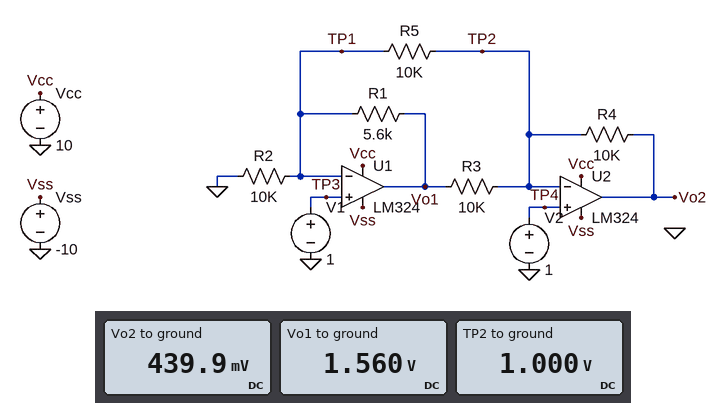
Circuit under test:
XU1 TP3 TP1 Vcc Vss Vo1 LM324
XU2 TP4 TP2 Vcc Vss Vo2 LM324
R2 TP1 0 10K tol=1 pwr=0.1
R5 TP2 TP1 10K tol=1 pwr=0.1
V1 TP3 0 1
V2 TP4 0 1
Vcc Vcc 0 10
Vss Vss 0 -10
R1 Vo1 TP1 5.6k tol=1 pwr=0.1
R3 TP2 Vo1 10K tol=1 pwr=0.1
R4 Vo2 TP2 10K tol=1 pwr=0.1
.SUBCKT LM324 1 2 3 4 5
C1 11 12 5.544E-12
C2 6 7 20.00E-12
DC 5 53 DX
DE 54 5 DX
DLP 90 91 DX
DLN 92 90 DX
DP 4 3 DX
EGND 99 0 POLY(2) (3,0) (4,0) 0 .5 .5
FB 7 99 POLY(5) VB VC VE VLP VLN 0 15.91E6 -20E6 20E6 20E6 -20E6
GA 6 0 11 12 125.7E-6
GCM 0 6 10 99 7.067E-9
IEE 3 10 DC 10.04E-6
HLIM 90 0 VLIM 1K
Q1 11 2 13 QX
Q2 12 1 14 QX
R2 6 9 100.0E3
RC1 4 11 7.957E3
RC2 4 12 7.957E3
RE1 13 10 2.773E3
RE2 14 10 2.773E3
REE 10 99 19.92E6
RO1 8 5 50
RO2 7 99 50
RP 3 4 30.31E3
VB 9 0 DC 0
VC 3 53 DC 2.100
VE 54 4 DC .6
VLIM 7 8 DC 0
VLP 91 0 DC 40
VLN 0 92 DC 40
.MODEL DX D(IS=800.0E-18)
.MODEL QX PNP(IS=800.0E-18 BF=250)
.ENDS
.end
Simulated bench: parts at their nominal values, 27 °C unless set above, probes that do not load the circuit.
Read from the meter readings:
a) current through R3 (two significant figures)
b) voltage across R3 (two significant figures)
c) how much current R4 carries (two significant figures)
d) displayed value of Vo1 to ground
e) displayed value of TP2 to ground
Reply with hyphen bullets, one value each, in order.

- 56 µA
- 560 mV
- 56 µA
- 1.560 V
- 1.000 V
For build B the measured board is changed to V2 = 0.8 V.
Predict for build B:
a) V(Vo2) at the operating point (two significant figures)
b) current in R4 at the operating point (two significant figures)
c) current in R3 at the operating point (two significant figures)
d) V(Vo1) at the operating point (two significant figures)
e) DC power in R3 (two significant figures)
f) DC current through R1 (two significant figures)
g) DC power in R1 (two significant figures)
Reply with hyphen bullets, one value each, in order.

- -270 mV
- 110 µA
- 87 µA
- 1.7 V
- 76 µW
- 120 µA
- 81 µW
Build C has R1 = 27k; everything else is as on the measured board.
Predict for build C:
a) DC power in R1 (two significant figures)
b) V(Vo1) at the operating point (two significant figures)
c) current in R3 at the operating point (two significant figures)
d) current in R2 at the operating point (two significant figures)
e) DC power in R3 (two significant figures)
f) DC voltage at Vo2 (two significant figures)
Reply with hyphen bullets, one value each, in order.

- 270 µW
- 3.7 V
- 270 µA
- 100 µA
- 730 µW
- -1.7 V
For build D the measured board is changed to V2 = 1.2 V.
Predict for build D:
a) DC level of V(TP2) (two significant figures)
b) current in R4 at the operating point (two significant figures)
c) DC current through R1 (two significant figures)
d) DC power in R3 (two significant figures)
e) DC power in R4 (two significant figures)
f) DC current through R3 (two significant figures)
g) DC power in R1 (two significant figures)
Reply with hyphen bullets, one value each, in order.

- 1.2 V
- 4.8 µA
- 80 µA
- 6.1 µW
- 230 nW
- 25 µA
- 36 µW
